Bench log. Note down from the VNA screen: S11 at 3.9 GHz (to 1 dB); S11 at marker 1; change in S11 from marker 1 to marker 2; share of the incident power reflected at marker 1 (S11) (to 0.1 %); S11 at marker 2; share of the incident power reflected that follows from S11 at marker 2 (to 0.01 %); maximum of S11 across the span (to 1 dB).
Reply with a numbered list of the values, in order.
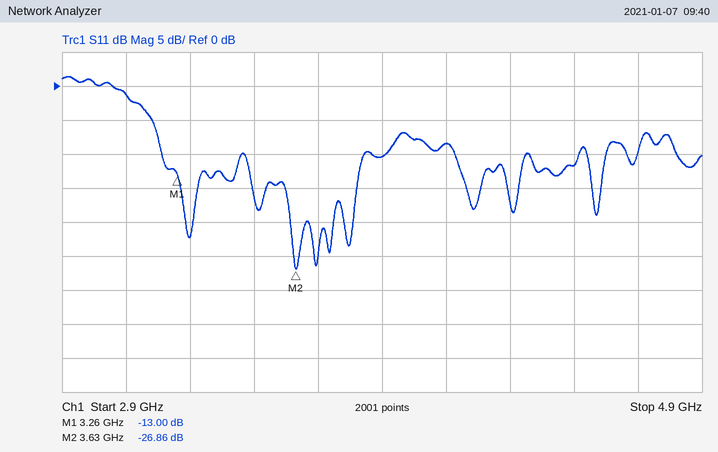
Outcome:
1. -10 dB
2. -13.00 dB
3. -13.86 dB
4. 5.0 %
5. -26.86 dB
6. 0.21 %
7. 1 dB
